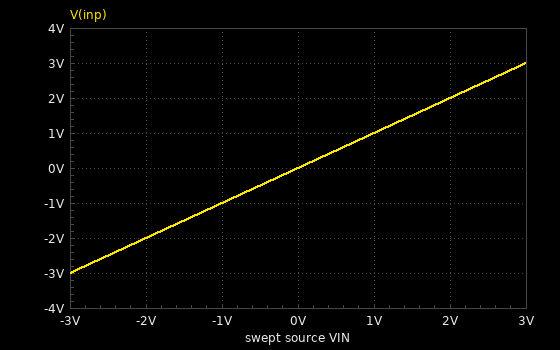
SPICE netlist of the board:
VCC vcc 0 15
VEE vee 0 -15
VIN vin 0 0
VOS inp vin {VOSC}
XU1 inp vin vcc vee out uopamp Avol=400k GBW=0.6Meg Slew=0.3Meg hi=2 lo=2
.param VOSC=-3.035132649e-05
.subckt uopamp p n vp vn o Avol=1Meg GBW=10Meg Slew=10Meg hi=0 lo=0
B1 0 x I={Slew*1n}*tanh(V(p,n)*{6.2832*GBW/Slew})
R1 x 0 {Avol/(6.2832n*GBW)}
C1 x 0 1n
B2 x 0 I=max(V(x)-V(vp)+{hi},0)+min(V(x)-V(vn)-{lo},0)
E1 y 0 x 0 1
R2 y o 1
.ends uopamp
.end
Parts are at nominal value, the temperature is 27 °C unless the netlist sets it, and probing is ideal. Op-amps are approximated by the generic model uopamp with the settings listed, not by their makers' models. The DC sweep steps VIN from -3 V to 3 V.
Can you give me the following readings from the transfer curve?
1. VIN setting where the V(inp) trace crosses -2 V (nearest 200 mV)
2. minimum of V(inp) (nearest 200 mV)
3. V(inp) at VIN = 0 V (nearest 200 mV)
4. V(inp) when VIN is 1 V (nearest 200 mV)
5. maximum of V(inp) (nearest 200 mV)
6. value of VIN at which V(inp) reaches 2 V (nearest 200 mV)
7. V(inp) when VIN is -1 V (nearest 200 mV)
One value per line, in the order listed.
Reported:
-2.0 V
-3.0 V
0 V
1.0 V
3.0 V
2.0 V
-1.0 V
